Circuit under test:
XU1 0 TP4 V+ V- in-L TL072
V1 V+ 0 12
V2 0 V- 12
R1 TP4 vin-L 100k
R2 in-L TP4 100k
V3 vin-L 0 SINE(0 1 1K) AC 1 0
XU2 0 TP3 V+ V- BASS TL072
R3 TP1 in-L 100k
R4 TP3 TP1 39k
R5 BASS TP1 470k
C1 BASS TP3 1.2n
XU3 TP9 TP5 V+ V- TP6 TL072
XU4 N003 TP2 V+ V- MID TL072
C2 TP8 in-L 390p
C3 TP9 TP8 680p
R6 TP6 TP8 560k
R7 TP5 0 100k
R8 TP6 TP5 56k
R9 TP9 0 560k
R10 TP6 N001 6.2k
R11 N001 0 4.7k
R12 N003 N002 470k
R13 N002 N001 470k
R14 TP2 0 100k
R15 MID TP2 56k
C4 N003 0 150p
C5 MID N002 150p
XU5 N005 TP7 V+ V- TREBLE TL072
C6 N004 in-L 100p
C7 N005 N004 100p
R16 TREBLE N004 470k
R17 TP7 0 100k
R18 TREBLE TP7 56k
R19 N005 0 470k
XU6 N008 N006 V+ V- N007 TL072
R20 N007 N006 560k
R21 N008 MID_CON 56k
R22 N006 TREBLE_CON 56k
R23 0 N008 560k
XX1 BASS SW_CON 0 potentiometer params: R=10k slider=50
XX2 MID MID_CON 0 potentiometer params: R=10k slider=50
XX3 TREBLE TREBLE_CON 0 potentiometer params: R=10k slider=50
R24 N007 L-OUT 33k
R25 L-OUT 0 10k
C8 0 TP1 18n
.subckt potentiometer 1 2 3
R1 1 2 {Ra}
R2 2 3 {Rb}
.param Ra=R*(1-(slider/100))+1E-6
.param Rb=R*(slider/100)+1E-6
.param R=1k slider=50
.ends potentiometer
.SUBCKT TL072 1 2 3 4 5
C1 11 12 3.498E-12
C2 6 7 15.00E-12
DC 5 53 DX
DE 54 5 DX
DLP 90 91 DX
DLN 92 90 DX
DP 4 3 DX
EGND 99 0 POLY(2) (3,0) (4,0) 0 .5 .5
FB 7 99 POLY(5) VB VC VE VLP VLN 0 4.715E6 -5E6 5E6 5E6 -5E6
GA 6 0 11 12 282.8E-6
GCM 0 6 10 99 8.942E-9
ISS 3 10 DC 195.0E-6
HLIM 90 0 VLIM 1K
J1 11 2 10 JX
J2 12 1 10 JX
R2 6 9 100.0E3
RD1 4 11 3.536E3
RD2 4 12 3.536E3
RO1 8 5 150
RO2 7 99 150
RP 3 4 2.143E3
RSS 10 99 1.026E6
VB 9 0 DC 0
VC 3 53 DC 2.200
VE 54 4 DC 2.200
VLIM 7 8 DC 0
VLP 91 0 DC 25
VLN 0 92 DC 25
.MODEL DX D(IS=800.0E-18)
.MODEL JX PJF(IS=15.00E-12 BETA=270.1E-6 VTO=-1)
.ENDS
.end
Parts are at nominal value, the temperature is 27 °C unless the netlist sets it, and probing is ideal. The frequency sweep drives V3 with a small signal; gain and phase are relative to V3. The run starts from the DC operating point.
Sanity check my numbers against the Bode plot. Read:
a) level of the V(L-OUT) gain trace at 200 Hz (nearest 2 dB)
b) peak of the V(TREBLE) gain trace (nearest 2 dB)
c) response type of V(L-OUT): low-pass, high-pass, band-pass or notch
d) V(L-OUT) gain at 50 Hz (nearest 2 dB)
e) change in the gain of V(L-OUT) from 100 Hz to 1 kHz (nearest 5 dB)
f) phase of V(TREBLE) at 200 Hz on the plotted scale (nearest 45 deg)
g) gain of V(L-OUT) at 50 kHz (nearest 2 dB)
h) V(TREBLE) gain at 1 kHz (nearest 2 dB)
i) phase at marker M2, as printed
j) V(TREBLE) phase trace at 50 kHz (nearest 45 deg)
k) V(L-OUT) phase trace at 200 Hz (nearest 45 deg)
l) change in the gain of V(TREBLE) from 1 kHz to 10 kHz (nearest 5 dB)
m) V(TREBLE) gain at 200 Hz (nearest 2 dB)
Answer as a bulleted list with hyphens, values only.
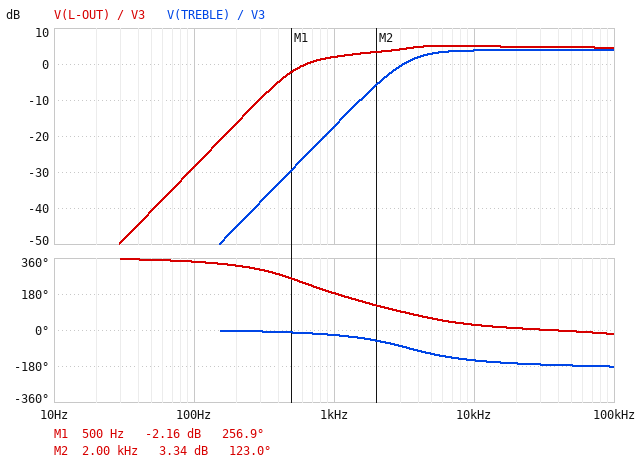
- -16 dB
- 4 dB
- high-pass
- -40 dB
- 30 dB
- 0 deg
- 4 dB
- -18 dB
- 123.0 deg
- -180 deg
- 315 deg
- 20 dB
- -46 dB
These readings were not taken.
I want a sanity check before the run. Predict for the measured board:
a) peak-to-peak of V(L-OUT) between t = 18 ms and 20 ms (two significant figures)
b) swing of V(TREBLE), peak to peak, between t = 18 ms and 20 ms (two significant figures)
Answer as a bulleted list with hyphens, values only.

- 2.5 V
- 270 mV
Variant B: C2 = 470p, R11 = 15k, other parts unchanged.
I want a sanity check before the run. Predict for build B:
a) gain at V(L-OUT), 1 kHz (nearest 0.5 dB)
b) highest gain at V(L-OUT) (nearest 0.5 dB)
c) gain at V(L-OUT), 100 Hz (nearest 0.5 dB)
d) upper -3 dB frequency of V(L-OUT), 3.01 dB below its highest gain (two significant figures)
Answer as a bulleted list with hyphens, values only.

- 6.0 dB
- 6.5 dB
- -22.5 dB
- 210 kHz
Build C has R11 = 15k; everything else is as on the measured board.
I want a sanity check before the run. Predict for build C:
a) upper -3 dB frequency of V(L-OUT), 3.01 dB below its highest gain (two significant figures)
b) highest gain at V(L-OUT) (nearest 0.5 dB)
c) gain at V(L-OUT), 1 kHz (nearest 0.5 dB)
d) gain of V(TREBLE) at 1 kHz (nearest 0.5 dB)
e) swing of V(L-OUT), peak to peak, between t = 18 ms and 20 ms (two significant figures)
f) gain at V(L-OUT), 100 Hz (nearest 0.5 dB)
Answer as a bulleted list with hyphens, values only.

- 210 kHz
- 6.5 dB
- 6.0 dB
- -17.5 dB
- 3.9 V
- -24.0 dB
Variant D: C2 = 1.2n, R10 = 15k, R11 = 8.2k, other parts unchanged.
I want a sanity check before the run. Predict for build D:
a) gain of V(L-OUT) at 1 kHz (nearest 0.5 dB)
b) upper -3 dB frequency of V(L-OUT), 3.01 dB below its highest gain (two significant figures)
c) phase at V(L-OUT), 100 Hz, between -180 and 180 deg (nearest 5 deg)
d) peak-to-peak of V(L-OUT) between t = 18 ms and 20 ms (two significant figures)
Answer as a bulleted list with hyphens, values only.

- 0.5 dB
- 320 kHz
- -35 deg
- 2.1 V
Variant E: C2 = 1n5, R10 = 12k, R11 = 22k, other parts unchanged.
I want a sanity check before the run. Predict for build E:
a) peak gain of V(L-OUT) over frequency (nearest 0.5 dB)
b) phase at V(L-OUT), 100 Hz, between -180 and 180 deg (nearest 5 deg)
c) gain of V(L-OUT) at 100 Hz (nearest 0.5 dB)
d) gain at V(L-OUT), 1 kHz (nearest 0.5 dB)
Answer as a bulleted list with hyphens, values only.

- 5.5 dB
- -40 deg
- -14.0 dB
- 5.0 dB
